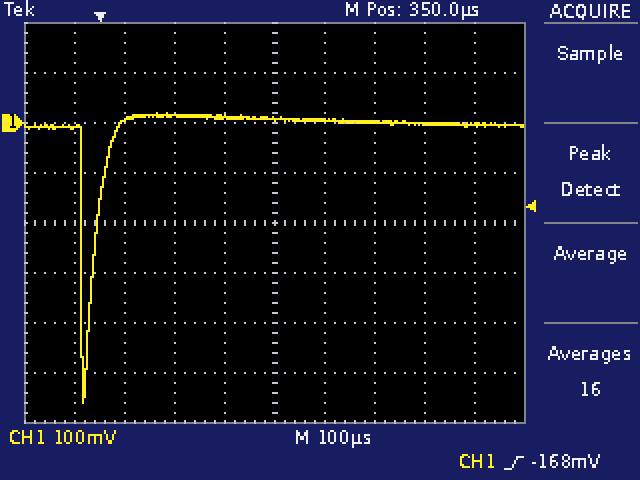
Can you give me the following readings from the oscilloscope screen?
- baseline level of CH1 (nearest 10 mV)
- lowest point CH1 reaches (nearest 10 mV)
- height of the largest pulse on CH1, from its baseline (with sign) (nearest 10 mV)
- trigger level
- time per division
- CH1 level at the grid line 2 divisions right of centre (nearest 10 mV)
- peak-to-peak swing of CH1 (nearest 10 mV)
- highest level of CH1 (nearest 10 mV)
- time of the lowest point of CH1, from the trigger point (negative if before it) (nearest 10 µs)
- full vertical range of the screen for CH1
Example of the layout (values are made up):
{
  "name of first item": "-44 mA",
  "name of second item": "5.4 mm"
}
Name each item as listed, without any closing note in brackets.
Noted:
{
  "baseline level of CH1": "0 mV",
  "lowest point CH1 reaches": "-560 mV",
  "height of the largest pulse on CH1, from its baseline (with sign)": "-560 mV",
  "trigger level": "-168 mV",
  "time per division": "100 µs",
  "CH1 level at the grid line 2 divisions right of centre": "0 mV",
  "peak-to-peak swing of CH1": "580 mV",
  "highest level of CH1": "20 mV",
  "time of the lowest point of CH1, from the trigger point (negative if before it)": "-30 µs",
  "full vertical range of the screen for CH1": "800 mV"
}
